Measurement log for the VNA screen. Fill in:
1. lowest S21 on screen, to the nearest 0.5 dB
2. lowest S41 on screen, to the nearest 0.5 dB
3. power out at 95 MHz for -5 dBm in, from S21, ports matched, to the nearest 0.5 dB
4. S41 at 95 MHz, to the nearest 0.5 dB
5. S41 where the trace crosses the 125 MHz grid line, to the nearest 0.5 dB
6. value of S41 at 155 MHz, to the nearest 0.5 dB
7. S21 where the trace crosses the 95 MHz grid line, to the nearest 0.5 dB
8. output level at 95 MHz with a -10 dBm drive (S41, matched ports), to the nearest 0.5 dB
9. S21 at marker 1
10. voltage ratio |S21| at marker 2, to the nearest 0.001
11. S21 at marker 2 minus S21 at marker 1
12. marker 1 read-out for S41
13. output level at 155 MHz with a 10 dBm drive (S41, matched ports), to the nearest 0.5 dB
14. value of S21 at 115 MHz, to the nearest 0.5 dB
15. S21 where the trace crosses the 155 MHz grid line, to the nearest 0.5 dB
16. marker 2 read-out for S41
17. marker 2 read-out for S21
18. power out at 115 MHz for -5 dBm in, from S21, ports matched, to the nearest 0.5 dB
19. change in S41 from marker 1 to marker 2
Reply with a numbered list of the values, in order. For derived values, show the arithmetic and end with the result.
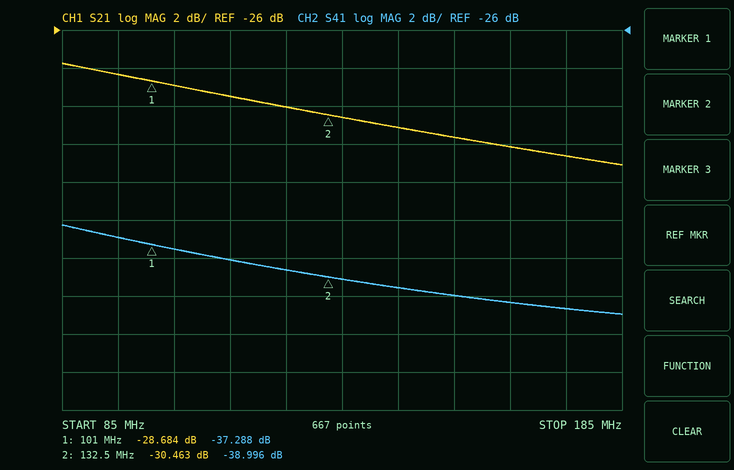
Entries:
1. -33.0 dB
2. -41.0 dB
3. -5 dBm + (-28.5 dB) = -33.5 dBm
4. -37.0 dB
5. -38.5 dB
6. -40.0 dB
7. -28.5 dB
8. -10 dBm + (-37.0 dB) = -47.0 dBm
9. -28.684 dB
10. 10^(-30.463/20) ≈ 0.030
11. -30.463 − (-28.684) = -1.779 dB
12. -37.288 dB
13. 10 dBm + (-40.0 dB) = -30.0 dBm
14. -29.5 dB
15. -31.5 dB
16. -38.996 dB
17. -30.463 dB
18. -5 dBm + (-29.5 dB) = -34.5 dBm
19. -38.996 − (-37.288) = -1.708 dB
